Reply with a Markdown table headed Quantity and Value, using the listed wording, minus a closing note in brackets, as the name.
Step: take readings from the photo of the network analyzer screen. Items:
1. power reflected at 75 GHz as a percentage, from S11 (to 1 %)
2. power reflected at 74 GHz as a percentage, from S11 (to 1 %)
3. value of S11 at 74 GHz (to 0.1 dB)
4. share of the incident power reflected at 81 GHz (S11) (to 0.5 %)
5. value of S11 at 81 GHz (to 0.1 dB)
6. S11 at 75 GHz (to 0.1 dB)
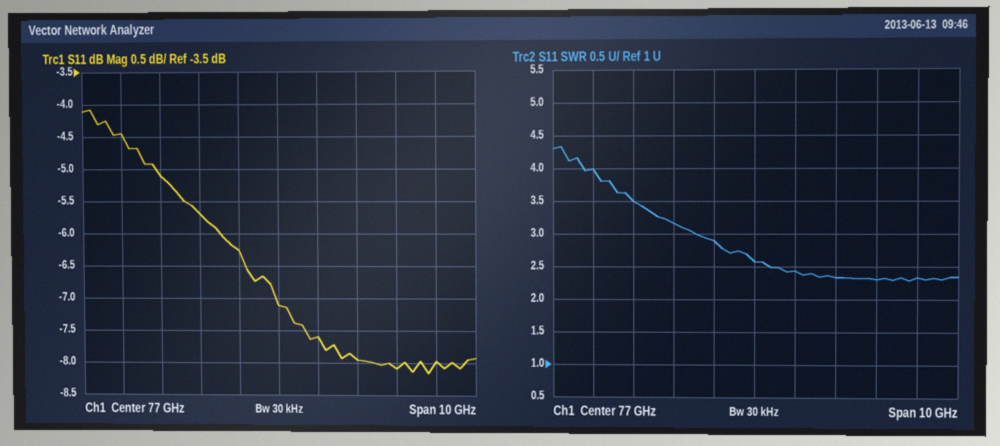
| Quantity | Value |
|---|---|
| power reflected at 75 GHz as a percentage, from S11 | 27 % |
| power reflected at 74 GHz as a percentage, from S11 | 31 % |
| value of S11 at 74 GHz | -5.1 dB |
| share of the incident power reflected at 81 GHz (S11) | 16.0 % |
| value of S11 at 81 GHz | -8.0 dB |
| S11 at 75 GHz | -5.7 dB |
